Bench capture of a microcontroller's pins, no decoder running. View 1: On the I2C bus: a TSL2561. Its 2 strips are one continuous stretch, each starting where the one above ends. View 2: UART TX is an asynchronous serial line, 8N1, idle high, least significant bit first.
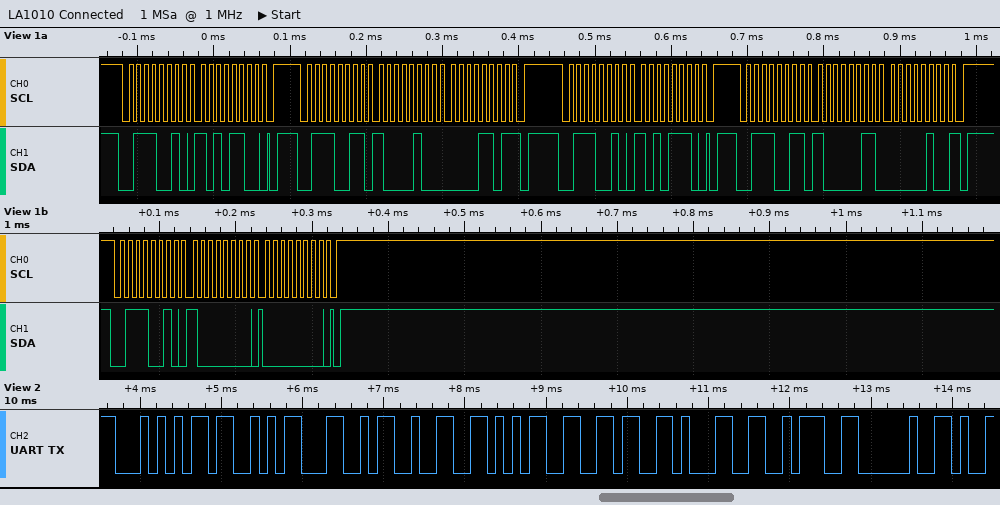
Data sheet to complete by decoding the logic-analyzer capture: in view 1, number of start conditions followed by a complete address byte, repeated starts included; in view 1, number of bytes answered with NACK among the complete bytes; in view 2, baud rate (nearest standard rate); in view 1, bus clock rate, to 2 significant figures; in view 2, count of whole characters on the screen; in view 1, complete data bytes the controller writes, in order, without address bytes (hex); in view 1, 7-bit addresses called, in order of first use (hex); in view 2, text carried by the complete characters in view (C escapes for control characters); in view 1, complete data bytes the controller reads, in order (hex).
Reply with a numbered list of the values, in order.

1. 5
2. 2
3. 9600 baud
4. 100 kHz
5. 9
6. AC AE 80 00
7. 0x39
8. "TSL2561: "
9. 84 0D 83 04
